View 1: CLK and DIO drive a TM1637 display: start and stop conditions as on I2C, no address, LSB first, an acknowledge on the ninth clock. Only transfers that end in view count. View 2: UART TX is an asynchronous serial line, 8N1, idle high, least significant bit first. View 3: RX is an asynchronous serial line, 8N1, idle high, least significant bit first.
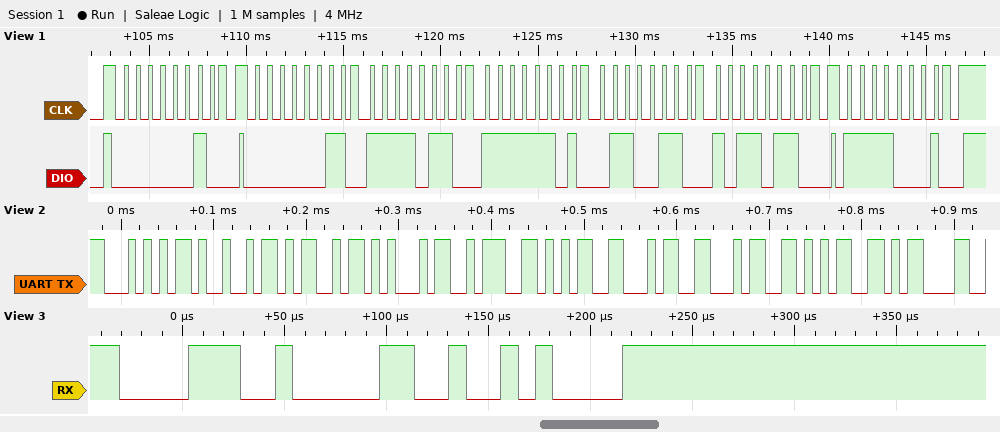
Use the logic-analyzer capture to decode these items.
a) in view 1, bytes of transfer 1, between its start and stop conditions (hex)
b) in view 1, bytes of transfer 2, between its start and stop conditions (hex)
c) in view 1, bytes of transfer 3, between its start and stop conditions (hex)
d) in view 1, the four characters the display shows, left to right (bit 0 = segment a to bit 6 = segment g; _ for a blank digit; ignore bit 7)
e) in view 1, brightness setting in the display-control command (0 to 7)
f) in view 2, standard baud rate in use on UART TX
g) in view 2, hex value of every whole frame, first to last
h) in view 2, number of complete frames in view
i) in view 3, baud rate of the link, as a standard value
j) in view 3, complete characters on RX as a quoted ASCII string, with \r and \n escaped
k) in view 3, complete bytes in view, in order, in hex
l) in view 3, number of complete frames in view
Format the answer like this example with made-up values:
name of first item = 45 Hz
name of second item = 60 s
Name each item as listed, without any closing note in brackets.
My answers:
in view 1, bytes of transfer 1, between its start and stop conditions = 40
in view 1, bytes of transfer 2, between its start and stop conditions = C0 6F BF 66 6D
in view 1, bytes of transfer 3, between its start and stop conditions = 8F
in view 1, the four characters the display shows, left to right = 9045
in view 1, brightness setting in the display-control command = 7
in view 2, standard baud rate in use on UART TX = 115200 baud
in view 2, hex value of every whole frame, first to last = 0x54 0x49 0x4D 0x45 0x3A 0x35 0x34 0x34 0x35 0x0D
in view 2, number of complete frames in view = 10
in view 3, baud rate of the link, as a standard value = 115200 baud
in view 3, complete characters on RX as a quoted ASCII string, with \r and \n escaped = "80\n"
in view 3, complete bytes in view, in order, in hex = 0x38 0x30 0x0A
in view 3, number of complete frames in view = 3
